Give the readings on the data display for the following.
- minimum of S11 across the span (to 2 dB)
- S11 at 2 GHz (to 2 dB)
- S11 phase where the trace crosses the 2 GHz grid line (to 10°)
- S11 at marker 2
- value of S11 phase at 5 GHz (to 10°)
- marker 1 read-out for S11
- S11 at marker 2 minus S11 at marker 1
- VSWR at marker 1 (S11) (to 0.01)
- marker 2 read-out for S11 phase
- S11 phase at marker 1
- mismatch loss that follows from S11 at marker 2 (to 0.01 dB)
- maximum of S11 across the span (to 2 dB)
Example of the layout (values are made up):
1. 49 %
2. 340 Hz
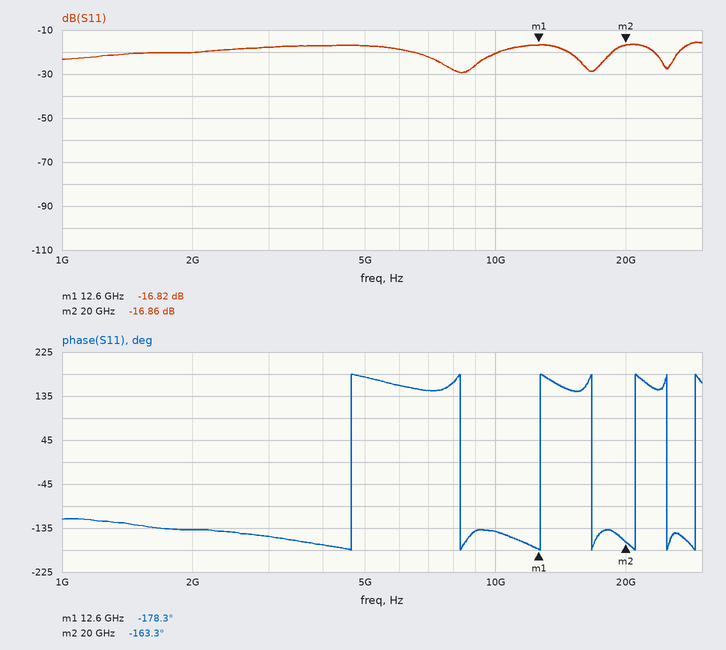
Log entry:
1. -30 dB
2. -20 dB
3. -140°
4. -16.86 dB
5. 170°
6. -16.82 dB
7. -0.04 dB
8. 1.34
9. -163.3°
10. -178.3°
11. 0.09 dB
12. -16 dB
